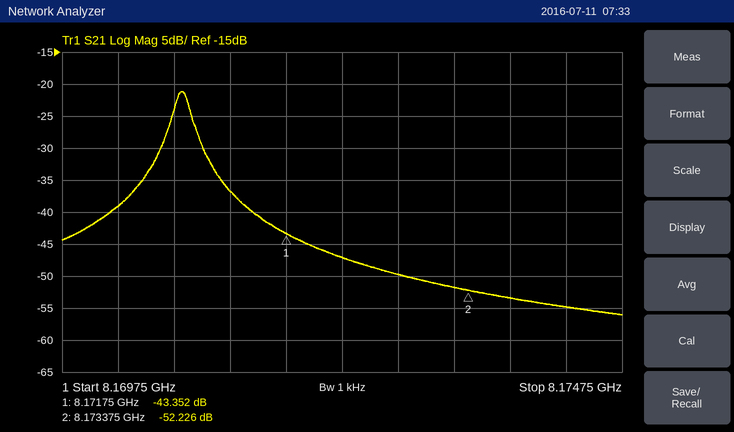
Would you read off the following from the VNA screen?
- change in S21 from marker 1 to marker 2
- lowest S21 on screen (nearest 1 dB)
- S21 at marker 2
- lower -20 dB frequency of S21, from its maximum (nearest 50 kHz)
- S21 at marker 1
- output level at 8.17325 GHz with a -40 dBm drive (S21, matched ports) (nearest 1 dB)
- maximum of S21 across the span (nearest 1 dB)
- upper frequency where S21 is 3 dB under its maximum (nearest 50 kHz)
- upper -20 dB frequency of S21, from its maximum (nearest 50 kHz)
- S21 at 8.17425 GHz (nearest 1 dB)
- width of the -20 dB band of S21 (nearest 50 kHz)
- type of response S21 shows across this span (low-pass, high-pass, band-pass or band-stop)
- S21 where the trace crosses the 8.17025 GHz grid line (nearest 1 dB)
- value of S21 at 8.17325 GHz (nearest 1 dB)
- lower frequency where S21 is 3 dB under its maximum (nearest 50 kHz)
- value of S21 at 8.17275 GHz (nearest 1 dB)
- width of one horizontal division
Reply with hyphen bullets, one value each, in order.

- -8.874 dB
- -56 dB
- -52.226 dB
- 8.17010 GHz
- -43.352 dB
- -92 dBm
- -21 dB
- 8.17090 GHz
- 8.17155 GHz
- -55 dB
- 1.45 MHz
- band-pass
- -39 dB
- -52 dB
- 8.17075 GHz
- -50 dB
- 500 kHz
